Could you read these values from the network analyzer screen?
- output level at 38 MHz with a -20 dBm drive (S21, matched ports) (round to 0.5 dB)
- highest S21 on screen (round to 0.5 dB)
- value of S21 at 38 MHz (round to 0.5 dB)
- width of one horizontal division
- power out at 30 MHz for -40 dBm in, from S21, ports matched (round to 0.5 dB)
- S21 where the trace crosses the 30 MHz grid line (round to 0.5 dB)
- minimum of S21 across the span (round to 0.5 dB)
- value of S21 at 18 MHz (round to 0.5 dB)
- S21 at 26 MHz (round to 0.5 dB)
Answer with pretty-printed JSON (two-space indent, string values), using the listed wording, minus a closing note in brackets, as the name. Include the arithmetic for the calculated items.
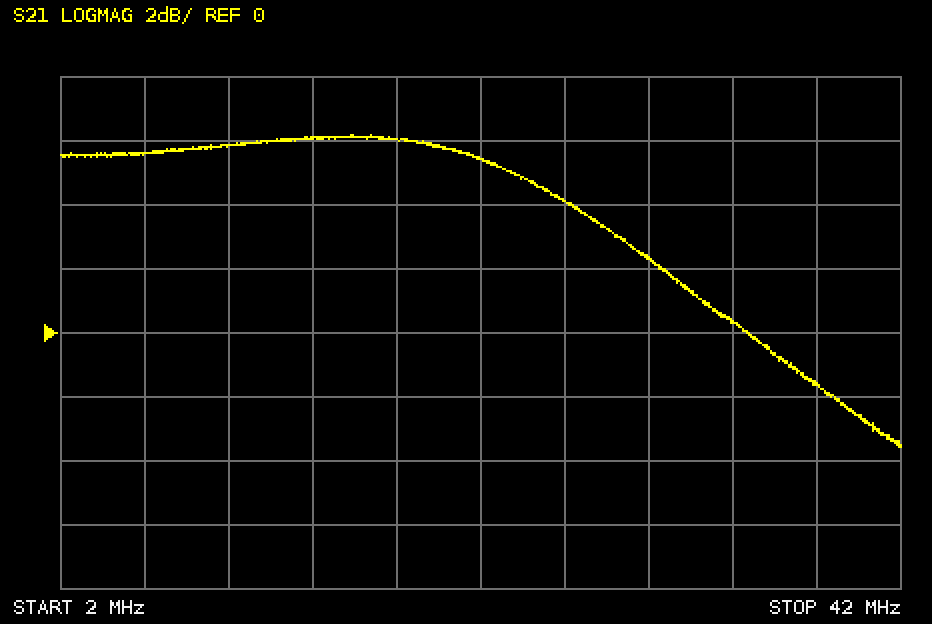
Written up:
{
  "output level at 38 MHz with a -20 dBm drive (S21, matched ports)": "-20 dBm + (-1.5 dB) = -21.5 dBm",
  "highest S21 on screen": "6.0 dB",
  "value of S21 at 38 MHz": "-1.5 dB",
  "width of one horizontal division": "4 MHz",
  "power out at 30 MHz for -40 dBm in, from S21, ports matched": "-40 dBm + (2.5 dB) = -37.5 dBm",
  "S21 where the trace crosses the 30 MHz grid line": "2.5 dB",
  "minimum of S21 across the span": "-3.5 dB",
  "value of S21 at 18 MHz": "6.0 dB",
  "S21 at 26 MHz": "4.0 dB"
}
